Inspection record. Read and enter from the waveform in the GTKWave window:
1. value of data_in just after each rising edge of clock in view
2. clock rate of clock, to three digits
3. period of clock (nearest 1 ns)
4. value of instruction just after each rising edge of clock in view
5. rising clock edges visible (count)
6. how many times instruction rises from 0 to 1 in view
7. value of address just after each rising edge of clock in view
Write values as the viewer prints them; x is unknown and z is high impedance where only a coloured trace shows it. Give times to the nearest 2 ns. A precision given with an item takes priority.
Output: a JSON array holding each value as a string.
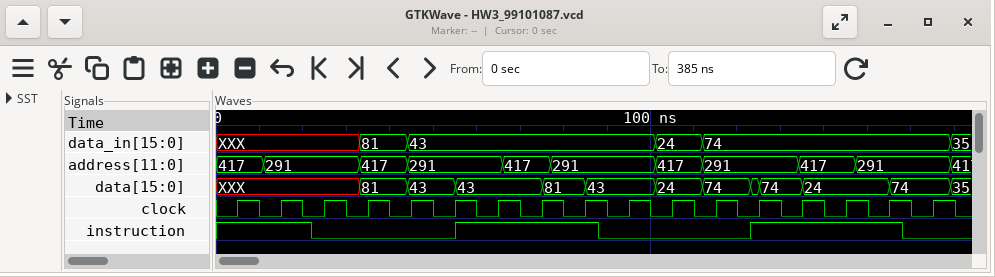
["XXX, XXX, XXX, 81, 43, 43, 43, 43, 43, 43, 24, 74, 74, 74, 74, 74, 74", "100 MHz", "10 ns", "1 1 0 0 0 1 1 1 1 0 0 0 1 1 1 1 0", "17", "2", "417, 291, 291, 417, 291, 291, 291, 417, 291, 291, 417, 291, 291, 417, 417, 291, 291"]
